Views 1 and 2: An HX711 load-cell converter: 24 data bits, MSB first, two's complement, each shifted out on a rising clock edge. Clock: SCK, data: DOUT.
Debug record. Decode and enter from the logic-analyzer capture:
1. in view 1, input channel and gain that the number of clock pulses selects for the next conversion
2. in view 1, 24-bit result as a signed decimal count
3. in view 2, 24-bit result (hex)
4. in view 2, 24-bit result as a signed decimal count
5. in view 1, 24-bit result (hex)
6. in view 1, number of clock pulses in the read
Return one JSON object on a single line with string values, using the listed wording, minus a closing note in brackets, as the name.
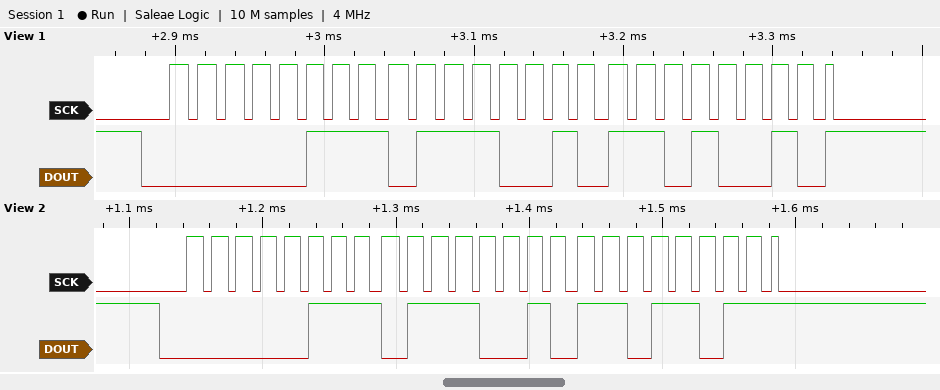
{"in view 1, input channel and gain that the number of clock pulses selects for the next conversion": "channel A, gain 128", "in view 1, 24-bit result as a signed decimal count": "488146", "in view 2, 24-bit result": "0x0772DB", "in view 2, 24-bit result as a signed decimal count": "488155", "in view 1, 24-bit result": "0x0772D2", "in view 1, number of clock pulses in the read": "25"}
